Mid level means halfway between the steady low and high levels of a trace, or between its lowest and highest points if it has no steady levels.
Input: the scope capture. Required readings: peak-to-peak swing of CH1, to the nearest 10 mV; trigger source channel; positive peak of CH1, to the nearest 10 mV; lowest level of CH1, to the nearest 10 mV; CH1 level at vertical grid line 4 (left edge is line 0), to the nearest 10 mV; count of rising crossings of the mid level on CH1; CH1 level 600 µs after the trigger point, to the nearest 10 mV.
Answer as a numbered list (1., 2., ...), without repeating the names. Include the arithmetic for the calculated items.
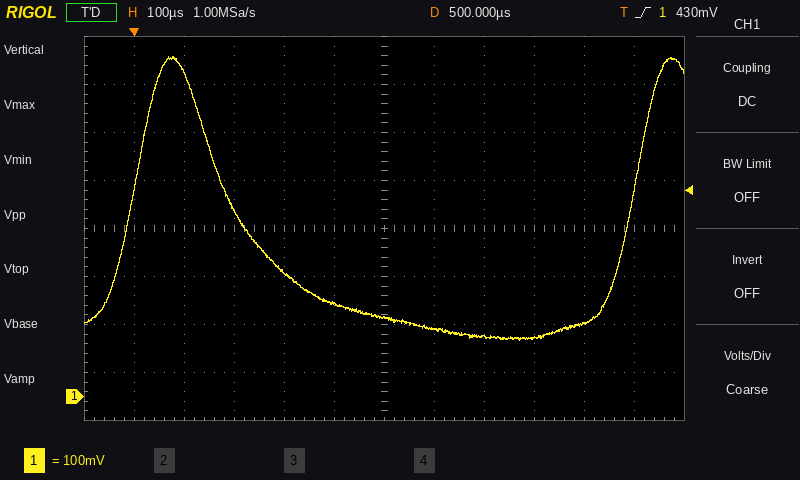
1. 710 mV − (120 mV) = 590 mV
2. CH1
3. 710 mV
4. 120 mV
5. 260 mV
6. 2
7. 140 mV
